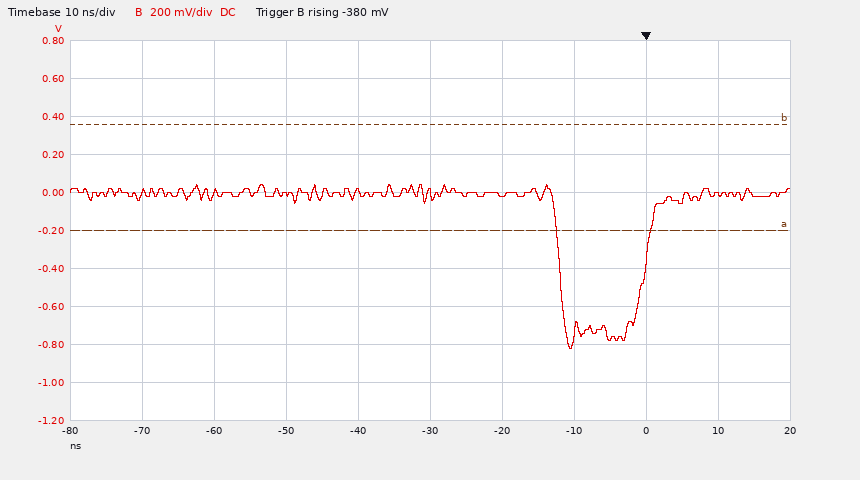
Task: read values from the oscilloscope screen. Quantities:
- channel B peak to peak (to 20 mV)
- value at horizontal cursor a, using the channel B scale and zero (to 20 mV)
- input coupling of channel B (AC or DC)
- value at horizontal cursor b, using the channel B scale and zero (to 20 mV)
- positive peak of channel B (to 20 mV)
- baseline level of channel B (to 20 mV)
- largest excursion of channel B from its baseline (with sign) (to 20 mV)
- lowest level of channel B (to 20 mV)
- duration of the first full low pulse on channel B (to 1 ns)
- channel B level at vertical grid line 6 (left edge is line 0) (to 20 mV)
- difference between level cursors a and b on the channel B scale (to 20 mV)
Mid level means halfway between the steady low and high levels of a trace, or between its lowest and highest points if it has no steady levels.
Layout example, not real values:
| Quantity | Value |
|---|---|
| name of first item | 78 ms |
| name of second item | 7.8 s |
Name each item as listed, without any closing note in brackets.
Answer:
| Quantity | Value |
|---|---|
| channel B peak to peak | 860 mV |
| value at horizontal cursor a, using the channel B scale and zero | -200 mV |
| input coupling of channel B | DC |
| value at horizontal cursor b, using the channel B scale and zero | 360 mV |
| positive peak of channel B | 40 mV |
| baseline level of channel B | 0 mV |
| largest excursion of channel B from its baseline (with sign) | -820 mV |
| lowest level of channel B | -820 mV |
| duration of the first full low pulse on channel B | 12 ns |
| channel B level at vertical grid line 6 (left edge is line 0) | -20 mV |
| difference between level cursors a and b on the channel B scale | 560 mV |
